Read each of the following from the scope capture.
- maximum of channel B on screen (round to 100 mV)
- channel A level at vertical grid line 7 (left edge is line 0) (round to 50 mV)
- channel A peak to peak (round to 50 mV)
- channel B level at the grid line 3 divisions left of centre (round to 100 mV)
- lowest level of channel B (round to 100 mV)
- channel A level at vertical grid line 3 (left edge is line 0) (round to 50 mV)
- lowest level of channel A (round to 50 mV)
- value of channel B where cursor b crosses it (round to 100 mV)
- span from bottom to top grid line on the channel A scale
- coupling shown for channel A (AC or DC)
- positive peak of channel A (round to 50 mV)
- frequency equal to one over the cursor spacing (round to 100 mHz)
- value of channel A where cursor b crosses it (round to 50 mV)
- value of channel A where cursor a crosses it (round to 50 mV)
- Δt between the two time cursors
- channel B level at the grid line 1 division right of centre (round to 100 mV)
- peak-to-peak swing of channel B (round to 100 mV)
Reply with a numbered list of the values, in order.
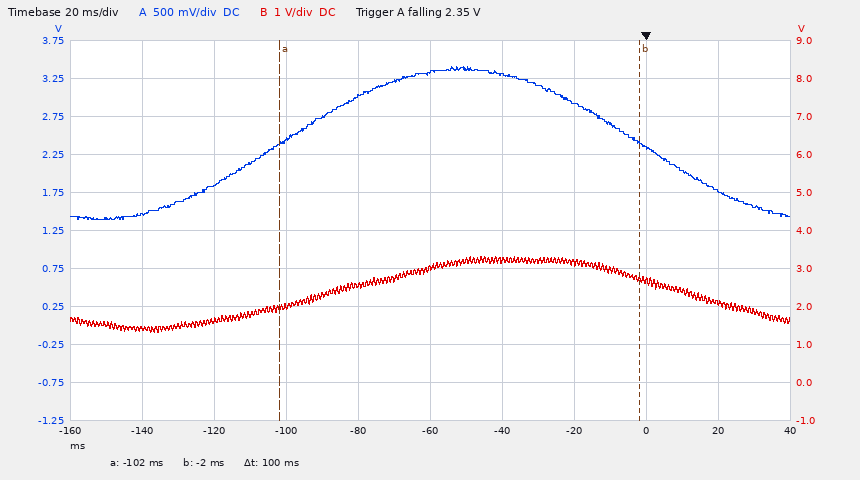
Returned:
1. 3.3 V
2. 2.95 V
3. 2.00 V
4. 1.6 V
5. 1.3 V
6. 2.45 V
7. 1.40 V
8. 2.7 V
9. 5 V
10. DC
11. 3.40 V
12. 10.0 Hz
13. 2.40 V
14. 2.40 V
15. 100 ms
16. 3.2 V
17. 2.0 V
